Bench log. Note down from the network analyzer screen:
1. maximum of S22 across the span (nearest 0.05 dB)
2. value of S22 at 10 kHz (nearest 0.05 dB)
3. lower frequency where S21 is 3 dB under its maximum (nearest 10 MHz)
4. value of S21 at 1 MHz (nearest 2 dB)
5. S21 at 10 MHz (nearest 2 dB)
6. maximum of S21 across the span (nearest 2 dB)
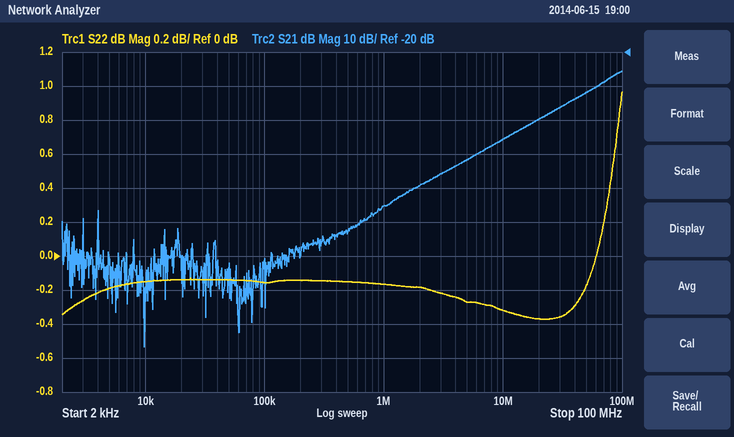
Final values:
0.95 dB
-0.15 dB
70 MHz
-66 dB
-46 dB
-26 dB
